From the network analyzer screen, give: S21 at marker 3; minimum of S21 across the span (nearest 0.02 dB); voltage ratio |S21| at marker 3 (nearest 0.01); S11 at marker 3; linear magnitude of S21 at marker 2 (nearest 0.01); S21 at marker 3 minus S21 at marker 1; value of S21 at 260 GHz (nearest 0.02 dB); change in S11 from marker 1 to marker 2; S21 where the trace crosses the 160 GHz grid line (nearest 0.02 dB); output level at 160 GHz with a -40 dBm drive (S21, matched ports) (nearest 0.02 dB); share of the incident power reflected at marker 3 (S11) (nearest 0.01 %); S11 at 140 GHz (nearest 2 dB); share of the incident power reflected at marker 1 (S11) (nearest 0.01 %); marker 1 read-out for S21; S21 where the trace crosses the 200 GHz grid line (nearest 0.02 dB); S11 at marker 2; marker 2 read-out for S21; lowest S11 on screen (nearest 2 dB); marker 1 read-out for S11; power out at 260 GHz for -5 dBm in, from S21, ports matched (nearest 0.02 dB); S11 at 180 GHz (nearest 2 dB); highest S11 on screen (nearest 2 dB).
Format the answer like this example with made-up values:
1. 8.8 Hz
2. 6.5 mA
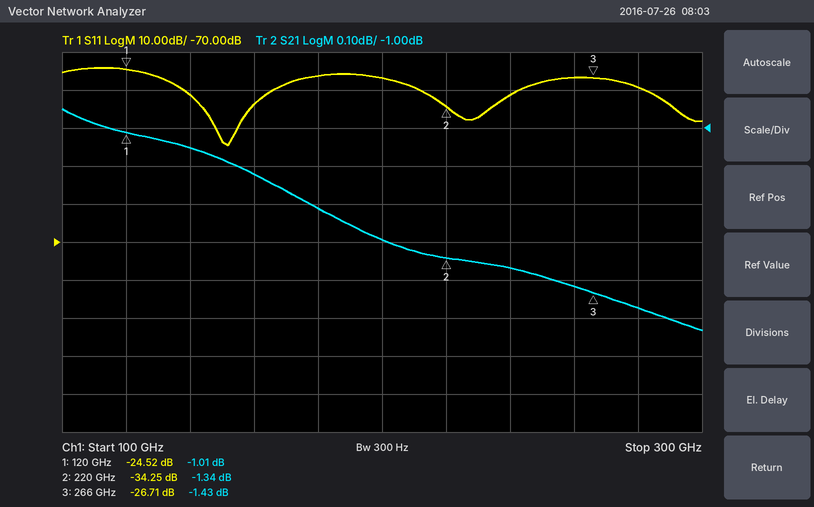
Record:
1. -1.43 dB
2. -1.54 dB
3. 0.85
4. -26.71 dB
5. 0.86
6. -0.42 dB
7. -1.42 dB
8. -9.73 dB
9. -1.12 dB
10. -41.12 dBm
11. 0.21 %
12. -32 dB
13. 0.35 %
14. -1.01 dB
15. -1.30 dB
16. -34.25 dB
17. -1.34 dB
18. -44 dB
19. -24.52 dB
20. -6.42 dBm
21. -26 dB
22. -24 dB
